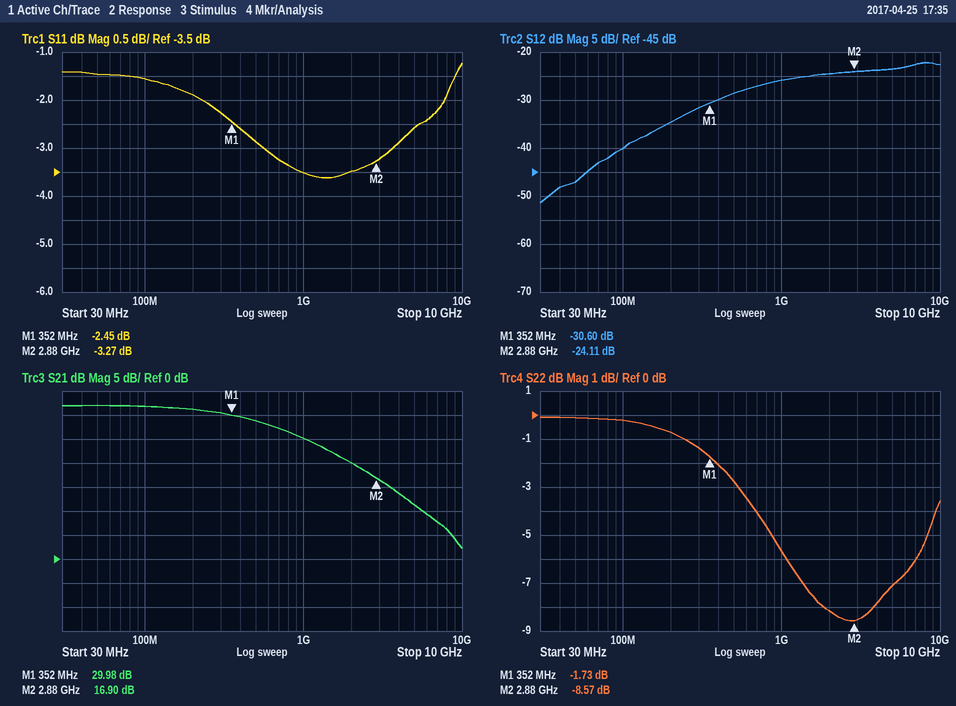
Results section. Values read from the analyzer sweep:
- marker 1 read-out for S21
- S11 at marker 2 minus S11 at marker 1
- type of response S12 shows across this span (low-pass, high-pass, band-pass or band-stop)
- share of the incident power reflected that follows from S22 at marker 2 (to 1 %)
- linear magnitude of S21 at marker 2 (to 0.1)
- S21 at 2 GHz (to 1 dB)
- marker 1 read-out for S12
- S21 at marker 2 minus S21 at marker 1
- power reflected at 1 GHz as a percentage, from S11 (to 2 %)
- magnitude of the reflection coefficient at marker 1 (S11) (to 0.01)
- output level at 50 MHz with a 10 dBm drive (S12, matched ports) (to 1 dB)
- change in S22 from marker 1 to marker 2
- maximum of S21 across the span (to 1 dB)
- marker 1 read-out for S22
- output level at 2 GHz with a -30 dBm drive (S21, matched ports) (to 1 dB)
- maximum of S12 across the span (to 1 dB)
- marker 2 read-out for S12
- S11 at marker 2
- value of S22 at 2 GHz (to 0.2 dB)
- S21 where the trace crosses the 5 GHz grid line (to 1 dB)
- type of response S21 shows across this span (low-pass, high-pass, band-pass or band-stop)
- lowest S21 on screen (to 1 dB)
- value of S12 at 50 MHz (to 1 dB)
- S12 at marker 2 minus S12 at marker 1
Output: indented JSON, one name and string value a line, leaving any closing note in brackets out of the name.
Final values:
{
  "marker 1 read-out for S21": "29.98 dB",
  "S11 at marker 2 minus S11 at marker 1": "-0.82 dB",
  "type of response S12 shows across this span": "high-pass",
  "share of the incident power reflected that follows from S22 at marker 2": "14 %",
  "linear magnitude of S21 at marker 2": "7.0",
  "S21 at 2 GHz": "20 dB",
  "marker 1 read-out for S12": "-30.60 dB",
  "S21 at marker 2 minus S21 at marker 1": "-13.08 dB",
  "power reflected at 1 GHz as a percentage, from S11": "44 %",
  "magnitude of the reflection coefficient at marker 1 (S11)": "0.75",
  "output level at 50 MHz with a 10 dBm drive (S12, matched ports)": "-37 dBm",
  "change in S22 from marker 1 to marker 2": "-6.84 dB",
  "maximum of S21 across the span": "32 dB",
  "marker 1 read-out for S22": "-1.73 dB",
  "output level at 2 GHz with a -30 dBm drive (S21, matched ports)": "-10 dBm",
  "maximum of S12 across the span": "-22 dB",
  "marker 2 read-out for S12": "-24.11 dB",
  "S11 at marker 2": "-3.27 dB",
  "value of S22 at 2 GHz": "-8.2 dB",
  "S21 where the trace crosses the 5 GHz grid line": "11 dB",
  "type of response S21 shows across this span": "low-pass",
  "lowest S21 on screen": "2 dB",
  "value of S12 at 50 MHz": "-47 dB",
  "S12 at marker 2 minus S12 at marker 1": "6.49 dB"
}
